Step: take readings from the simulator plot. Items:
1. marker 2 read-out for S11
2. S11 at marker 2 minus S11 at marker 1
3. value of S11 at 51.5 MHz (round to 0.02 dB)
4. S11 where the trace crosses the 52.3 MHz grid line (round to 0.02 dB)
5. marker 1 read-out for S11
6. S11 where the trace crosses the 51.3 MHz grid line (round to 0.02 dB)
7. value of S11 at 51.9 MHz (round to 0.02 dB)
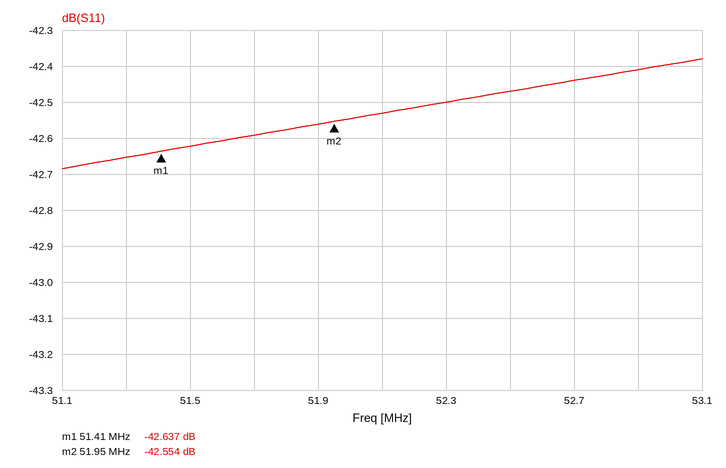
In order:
-42.554 dB
0.083 dB
-42.62 dB
-42.50 dB
-42.637 dB
-42.66 dB
-42.56 dB
